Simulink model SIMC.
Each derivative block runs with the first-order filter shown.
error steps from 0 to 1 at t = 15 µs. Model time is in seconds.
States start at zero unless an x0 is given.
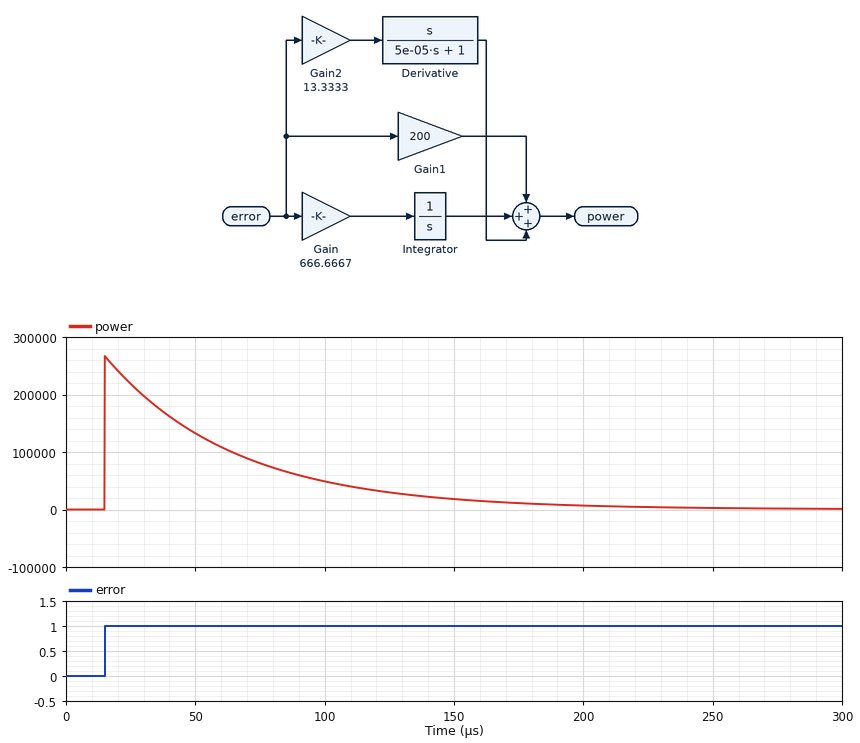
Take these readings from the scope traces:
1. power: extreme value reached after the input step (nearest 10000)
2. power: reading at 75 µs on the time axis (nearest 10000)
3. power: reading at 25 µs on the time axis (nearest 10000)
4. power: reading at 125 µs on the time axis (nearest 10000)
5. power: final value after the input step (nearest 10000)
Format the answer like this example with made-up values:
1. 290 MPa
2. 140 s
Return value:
1. 270000
2. 80000
3. 220000
4. 30000
5. 0
